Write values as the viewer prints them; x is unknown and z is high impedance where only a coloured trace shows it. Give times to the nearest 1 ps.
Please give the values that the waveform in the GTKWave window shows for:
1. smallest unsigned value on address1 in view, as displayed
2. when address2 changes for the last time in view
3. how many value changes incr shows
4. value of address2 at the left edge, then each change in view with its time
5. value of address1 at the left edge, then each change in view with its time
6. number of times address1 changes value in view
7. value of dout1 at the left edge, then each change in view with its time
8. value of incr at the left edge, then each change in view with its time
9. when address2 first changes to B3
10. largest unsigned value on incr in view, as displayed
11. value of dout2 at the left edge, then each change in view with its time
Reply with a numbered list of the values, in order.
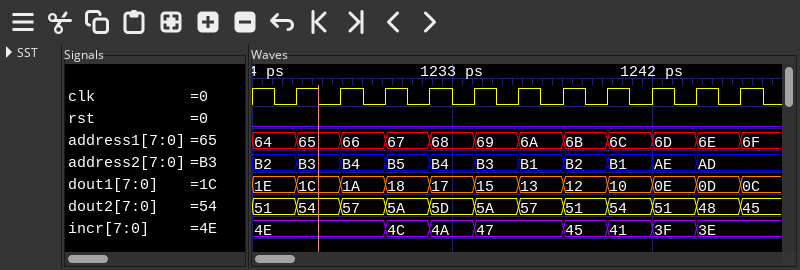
1. 64
2. 1244 ps
3. 7
4. B2, B3 at 1226 ps, B4 at 1228 ps, B5 at 1230 ps, B4 at 1232 ps, B3 at 1234 ps, B1 at 1236 ps, B2 at 1238 ps, B1 at 1240 ps, AE at 1242 ps, AD at 1244 ps
5. 64, 65 at 1226 ps, 66 at 1228 ps, 67 at 1230 ps, 68 at 1232 ps, 69 at 1234 ps, 6A at 1236 ps, 6B at 1238 ps, 6C at 1240 ps, 6D at 1242 ps, 6E at 1244 ps, 6F at 1246 ps
6. 11
7. 1E, 1C at 1226 ps, 1A at 1228 ps, 18 at 1230 ps, 17 at 1232 ps, 15 at 1234 ps, 13 at 1236 ps, 12 at 1238 ps, 10 at 1240 ps, 0E at 1242 ps, 0D at 1244 ps, 0C at 1246 ps
8. 4E, 4C at 1230 ps, 4A at 1232 ps, 47 at 1234 ps, 45 at 1238 ps, 41 at 1240 ps, 3F at 1242 ps, 3E at 1244 ps
9. 1226 ps
10. 4E
11. 51, 54 at 1226 ps, 57 at 1228 ps, 5A at 1230 ps, 5D at 1232 ps, 5A at 1234 ps, 57 at 1236 ps, 51 at 1238 ps, 54 at 1240 ps, 51 at 1242 ps, 48 at 1244 ps, 45 at 1246 ps
